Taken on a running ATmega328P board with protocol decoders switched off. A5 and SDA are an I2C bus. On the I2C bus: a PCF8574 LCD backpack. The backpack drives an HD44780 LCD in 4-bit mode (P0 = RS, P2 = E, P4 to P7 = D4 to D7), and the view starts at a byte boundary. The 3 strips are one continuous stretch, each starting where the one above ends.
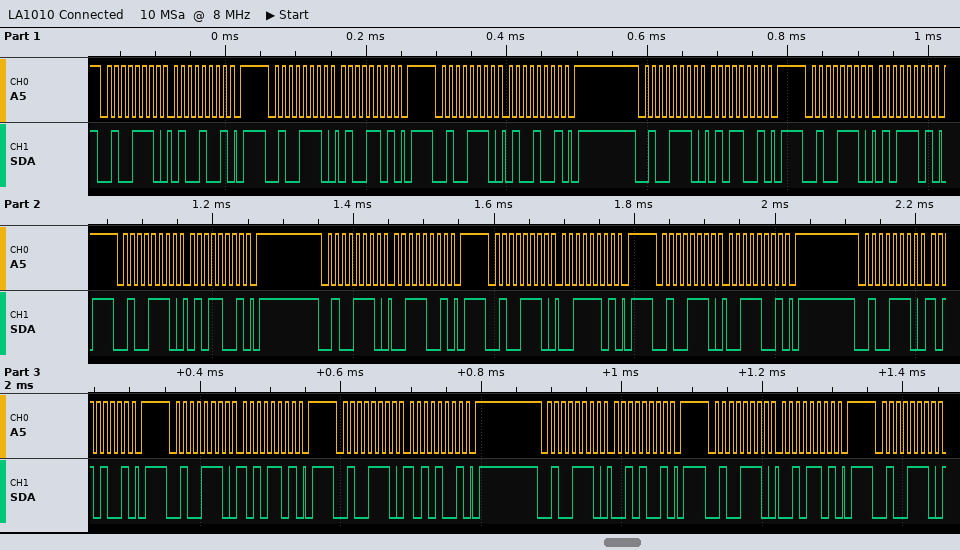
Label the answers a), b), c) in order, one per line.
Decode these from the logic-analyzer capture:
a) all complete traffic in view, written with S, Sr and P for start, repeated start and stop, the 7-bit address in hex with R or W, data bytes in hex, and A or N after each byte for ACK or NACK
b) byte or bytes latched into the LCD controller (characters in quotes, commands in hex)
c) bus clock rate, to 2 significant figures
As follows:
a) S 27W A 49 A P S 27W A 4D A P S 27W A 49 A P S 27W A 59 A P S 27W A 5D A P S 27W A 59 A P S 27W A 39 A P S 27W A 3D A P S 27W A 39 A P S 27W A A9 A P S 27W A AD A P S 27W A A9 A P S 27W A 29 A P S 27W A 2D A P S 27W A
b) 'E' ':'
c) 100 kHz
